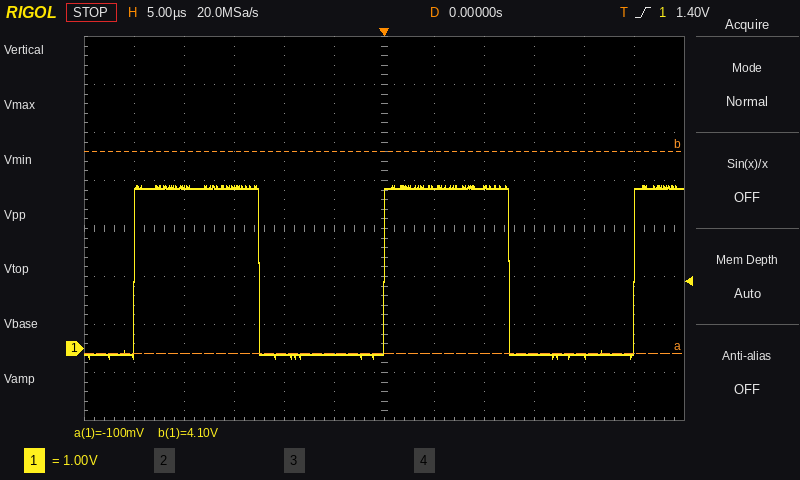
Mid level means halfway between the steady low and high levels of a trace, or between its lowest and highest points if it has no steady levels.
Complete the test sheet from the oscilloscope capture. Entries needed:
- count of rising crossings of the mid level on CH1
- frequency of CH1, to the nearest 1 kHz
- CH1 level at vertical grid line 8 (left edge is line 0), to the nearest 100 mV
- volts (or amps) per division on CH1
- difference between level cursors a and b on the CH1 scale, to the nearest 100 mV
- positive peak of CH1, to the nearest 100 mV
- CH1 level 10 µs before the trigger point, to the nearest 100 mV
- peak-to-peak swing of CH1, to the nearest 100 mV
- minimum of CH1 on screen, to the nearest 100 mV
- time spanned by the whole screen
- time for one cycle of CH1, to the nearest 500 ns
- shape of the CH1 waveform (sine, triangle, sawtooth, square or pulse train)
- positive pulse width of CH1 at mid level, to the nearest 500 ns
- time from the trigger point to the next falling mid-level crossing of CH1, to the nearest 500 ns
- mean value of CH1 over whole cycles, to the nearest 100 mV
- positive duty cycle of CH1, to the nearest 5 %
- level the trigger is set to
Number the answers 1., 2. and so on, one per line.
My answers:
1. 3
2. 40 kHz
3. 3.4 V
4. 1 V
5. 4.2 V
6. 3.4 V
7. -100 mV
8. 3.6 V
9. -200 mV
10. 60 µs
11. 25.0 µs
12. square
13. 12.5 µs
14. 12.5 µs
15. 1.6 V
16. 50 %
17. 1.40 V
